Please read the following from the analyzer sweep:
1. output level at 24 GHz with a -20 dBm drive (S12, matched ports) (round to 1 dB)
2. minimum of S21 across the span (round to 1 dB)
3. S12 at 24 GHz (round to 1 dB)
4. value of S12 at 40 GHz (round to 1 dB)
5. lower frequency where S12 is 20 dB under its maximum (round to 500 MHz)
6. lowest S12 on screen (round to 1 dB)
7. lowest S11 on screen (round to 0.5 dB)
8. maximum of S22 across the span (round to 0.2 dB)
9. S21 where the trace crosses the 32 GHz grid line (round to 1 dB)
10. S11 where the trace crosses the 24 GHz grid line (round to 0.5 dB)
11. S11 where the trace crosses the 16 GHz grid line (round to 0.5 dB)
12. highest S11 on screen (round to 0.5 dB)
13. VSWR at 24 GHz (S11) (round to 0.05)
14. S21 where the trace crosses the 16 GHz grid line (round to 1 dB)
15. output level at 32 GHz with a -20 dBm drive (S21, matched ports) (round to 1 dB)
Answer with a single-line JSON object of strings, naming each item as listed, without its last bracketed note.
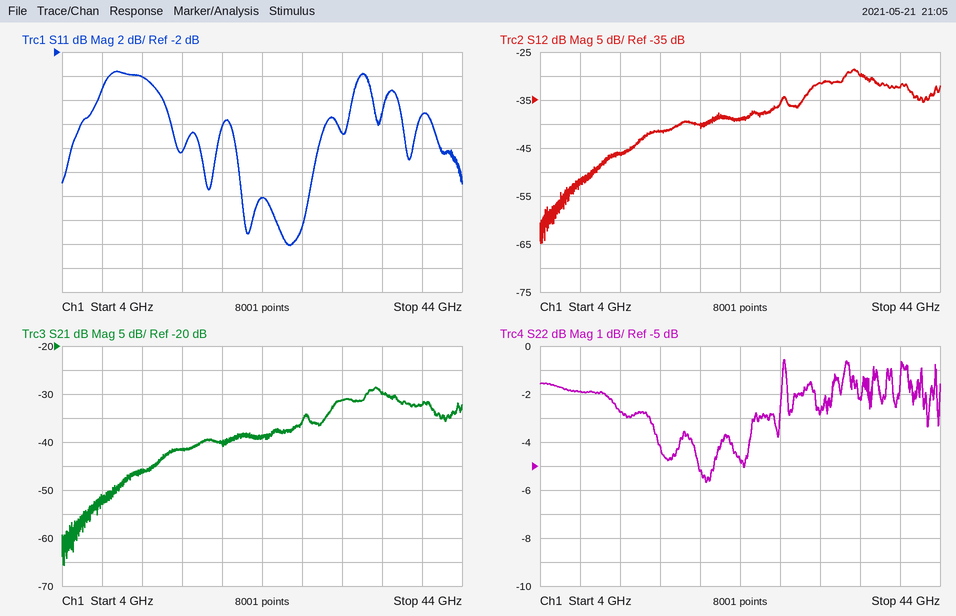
{"output level at 24 GHz with a -20 dBm drive (S12, matched ports)": "-59 dBm", "minimum of S21 across the span": "-66 dB", "S12 at 24 GHz": "-39 dB", "value of S12 at 40 GHz": "-32 dB", "lower frequency where S12 is 20 dB under its maximum": "10.0 GHz", "lowest S12 on screen": "-65 dB", "lowest S11 on screen": "-18.0 dB", "maximum of S22 across the span": "-0.6 dB", "S21 where the trace crosses the 32 GHz grid line": "-31 dB", "S11 where the trace crosses the 24 GHz grid line": "-14.0 dB", "S11 where the trace crosses the 16 GHz grid line": "-10.5 dB", "highest S11 on screen": "-3.5 dB", "VSWR at 24 GHz (S11)": "1.50", "S21 where the trace crosses the 16 GHz grid line": "-42 dB", "output level at 32 GHz with a -20 dBm drive (S21, matched ports)": "-51 dBm"}
